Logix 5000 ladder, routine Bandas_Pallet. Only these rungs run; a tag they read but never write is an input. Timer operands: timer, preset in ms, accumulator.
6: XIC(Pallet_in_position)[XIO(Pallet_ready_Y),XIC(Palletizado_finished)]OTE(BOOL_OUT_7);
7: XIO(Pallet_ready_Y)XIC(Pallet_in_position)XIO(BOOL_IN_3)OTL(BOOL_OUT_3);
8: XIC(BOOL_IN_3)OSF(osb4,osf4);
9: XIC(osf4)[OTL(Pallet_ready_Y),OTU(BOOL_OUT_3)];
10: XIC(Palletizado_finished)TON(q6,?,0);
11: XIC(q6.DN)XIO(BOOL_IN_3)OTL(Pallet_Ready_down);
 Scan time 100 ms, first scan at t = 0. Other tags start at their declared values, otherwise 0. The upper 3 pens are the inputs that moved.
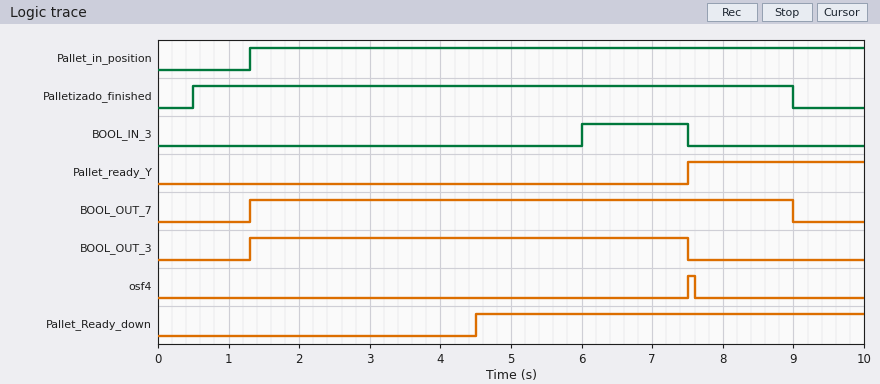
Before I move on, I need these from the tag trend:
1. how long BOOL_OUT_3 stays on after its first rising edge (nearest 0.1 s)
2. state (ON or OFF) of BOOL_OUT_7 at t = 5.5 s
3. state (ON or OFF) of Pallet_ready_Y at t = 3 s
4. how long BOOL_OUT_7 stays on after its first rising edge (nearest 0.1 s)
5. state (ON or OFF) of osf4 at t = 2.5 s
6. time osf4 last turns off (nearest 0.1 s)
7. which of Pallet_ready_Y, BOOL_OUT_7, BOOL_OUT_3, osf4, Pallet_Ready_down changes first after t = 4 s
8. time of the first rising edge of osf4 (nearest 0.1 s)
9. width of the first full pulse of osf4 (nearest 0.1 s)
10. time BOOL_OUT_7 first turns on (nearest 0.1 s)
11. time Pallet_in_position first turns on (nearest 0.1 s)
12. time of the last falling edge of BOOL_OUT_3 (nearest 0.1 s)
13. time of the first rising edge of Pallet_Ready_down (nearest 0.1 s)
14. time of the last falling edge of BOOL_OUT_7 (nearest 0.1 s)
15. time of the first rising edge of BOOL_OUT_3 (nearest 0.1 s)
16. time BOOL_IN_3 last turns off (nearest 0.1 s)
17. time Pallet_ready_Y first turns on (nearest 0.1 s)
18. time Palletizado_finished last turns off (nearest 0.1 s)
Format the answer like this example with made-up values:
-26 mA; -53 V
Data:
6.2 s; ON; OFF; 7.7 s; OFF; 7.6 s; Pallet_Ready_down; 7.5 s; 0.1 s; 1.3 s; 1.3 s; 7.5 s; 4.5 s; 9.0 s; 1.3 s; 7.5 s; 7.5 s; 9.0 s
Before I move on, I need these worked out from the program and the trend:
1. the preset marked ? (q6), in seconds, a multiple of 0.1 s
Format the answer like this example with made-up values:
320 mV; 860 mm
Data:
4.0 s
